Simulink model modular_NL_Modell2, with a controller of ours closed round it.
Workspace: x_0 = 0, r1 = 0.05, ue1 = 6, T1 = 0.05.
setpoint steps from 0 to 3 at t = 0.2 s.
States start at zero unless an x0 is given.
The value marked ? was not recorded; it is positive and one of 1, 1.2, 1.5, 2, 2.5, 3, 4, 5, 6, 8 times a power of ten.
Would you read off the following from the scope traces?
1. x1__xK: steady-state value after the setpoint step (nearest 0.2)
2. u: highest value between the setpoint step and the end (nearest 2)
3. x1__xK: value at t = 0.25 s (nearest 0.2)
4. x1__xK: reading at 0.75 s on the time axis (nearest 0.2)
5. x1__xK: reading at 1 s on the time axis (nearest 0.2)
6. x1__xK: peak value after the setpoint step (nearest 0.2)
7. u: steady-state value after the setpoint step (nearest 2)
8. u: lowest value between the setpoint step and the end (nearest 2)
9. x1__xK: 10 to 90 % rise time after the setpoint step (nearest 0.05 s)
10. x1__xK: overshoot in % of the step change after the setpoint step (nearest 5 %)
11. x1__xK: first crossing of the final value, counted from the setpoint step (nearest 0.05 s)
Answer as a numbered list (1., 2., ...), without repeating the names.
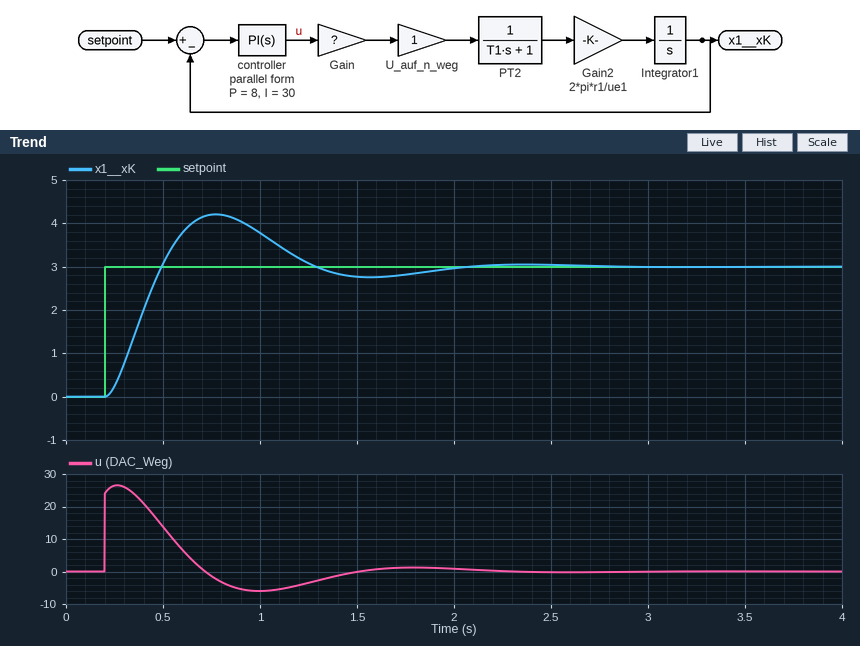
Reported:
1. 3.0
2. 26
3. 0.2
4. 4.2
5. 3.8
6. 4.2
7. 0
8. -6
9. 0.20 s
10. 40 %
11. 0.30 s
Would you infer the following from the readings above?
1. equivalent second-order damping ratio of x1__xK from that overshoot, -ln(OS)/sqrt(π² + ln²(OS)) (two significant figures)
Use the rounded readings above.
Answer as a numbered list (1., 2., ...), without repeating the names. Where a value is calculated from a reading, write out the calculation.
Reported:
1. ln(0.4) = -0.916; 0.916 / sqrt(9.870 + 0.840) = 0.28
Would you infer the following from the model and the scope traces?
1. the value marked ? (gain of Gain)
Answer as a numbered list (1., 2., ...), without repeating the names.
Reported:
1. 10
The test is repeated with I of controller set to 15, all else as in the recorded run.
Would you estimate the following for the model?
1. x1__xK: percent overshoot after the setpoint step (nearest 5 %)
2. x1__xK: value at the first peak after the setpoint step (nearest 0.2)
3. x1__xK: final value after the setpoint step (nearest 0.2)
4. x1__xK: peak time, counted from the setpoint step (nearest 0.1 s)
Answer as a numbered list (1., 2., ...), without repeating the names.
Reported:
1. 25 %
2. 3.8
3. 3.0
4. 0.7 s
